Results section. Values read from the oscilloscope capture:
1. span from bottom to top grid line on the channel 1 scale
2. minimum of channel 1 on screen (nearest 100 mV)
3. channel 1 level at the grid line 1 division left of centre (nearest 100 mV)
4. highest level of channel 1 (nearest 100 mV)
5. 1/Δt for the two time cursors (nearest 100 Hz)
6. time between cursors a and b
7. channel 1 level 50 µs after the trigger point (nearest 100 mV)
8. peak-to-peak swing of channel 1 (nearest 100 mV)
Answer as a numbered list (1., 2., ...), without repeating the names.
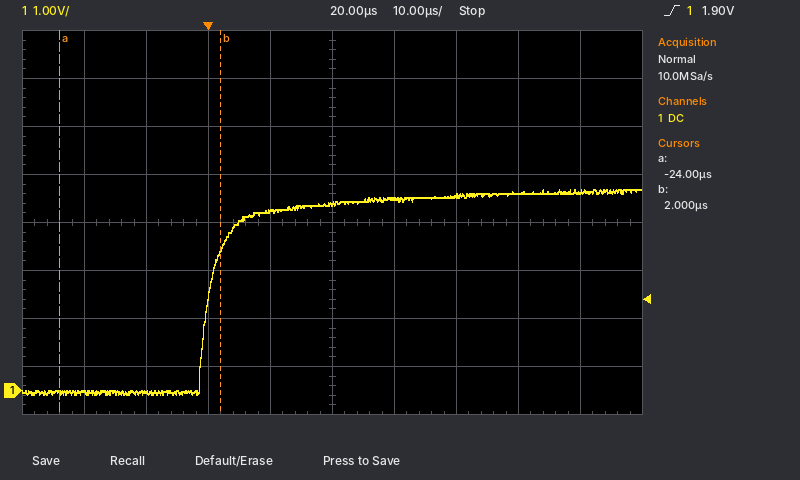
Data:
1. 8 V
2. -100 mV
3. 3.7 V
4. 4.2 V
5. 38.5 kHz
6. 26 µs
7. 4.1 V
8. 4.3 V
